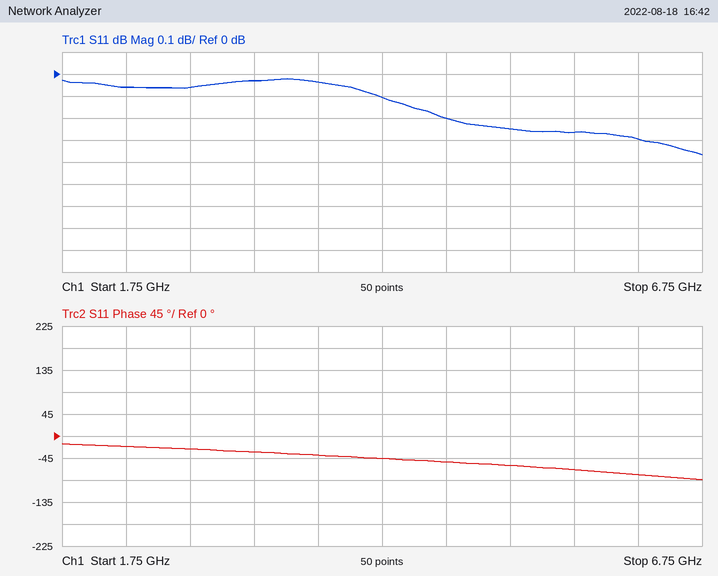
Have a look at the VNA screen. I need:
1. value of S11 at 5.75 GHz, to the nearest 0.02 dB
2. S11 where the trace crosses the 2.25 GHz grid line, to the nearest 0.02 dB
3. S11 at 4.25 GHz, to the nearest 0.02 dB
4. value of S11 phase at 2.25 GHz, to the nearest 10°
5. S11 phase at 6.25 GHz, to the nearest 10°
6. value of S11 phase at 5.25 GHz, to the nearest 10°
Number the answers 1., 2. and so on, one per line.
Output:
1. -0.26 dB
2. -0.06 dB
3. -0.10 dB
4. -20°
5. -80°
6. -60°
